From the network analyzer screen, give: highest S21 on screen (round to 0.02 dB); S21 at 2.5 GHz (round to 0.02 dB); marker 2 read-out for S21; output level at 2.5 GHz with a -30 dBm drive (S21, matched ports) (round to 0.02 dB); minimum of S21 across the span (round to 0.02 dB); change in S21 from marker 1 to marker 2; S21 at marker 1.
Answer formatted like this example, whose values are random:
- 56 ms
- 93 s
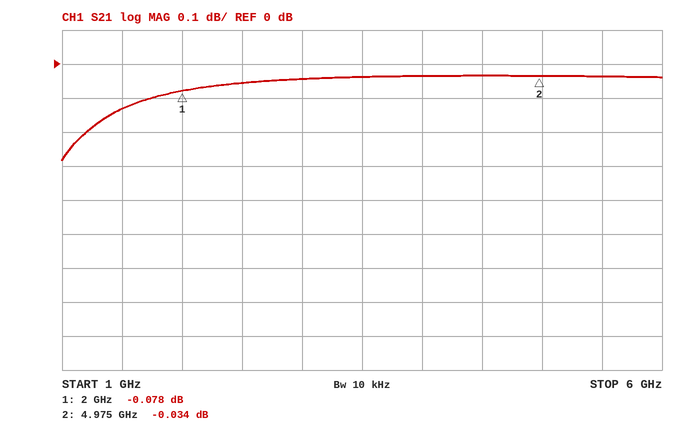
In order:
- -0.04 dB
- -0.06 dB
- -0.034 dB
- -30.06 dBm
- -0.28 dB
- 0.044 dB
- -0.078 dB
